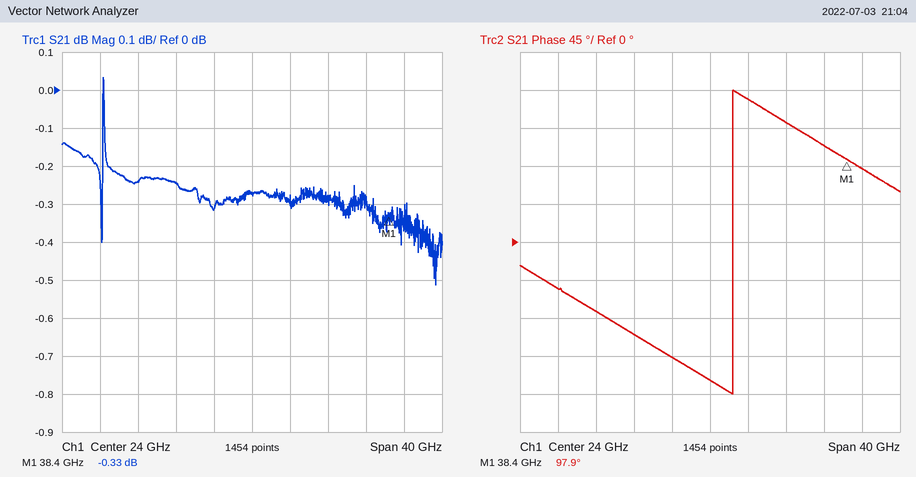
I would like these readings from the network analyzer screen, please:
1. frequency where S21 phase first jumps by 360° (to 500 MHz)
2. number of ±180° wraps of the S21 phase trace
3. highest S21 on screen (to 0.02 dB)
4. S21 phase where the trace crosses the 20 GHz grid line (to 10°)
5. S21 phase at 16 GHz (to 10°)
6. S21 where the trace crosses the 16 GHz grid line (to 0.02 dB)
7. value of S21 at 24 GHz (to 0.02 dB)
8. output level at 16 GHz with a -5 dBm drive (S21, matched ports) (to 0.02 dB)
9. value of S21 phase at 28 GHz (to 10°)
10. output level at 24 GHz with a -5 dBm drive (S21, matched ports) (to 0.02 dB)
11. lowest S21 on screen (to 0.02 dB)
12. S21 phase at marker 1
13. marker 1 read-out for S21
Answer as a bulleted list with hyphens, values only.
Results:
- 26.5 GHz
- 1
- 0.04 dB
- -140°
- -110°
- -0.24 dB
- -0.28 dB
- -5.24 dBm
- 170°
- -5.28 dBm
- -0.52 dB
- 97.9°
- -0.33 dB
